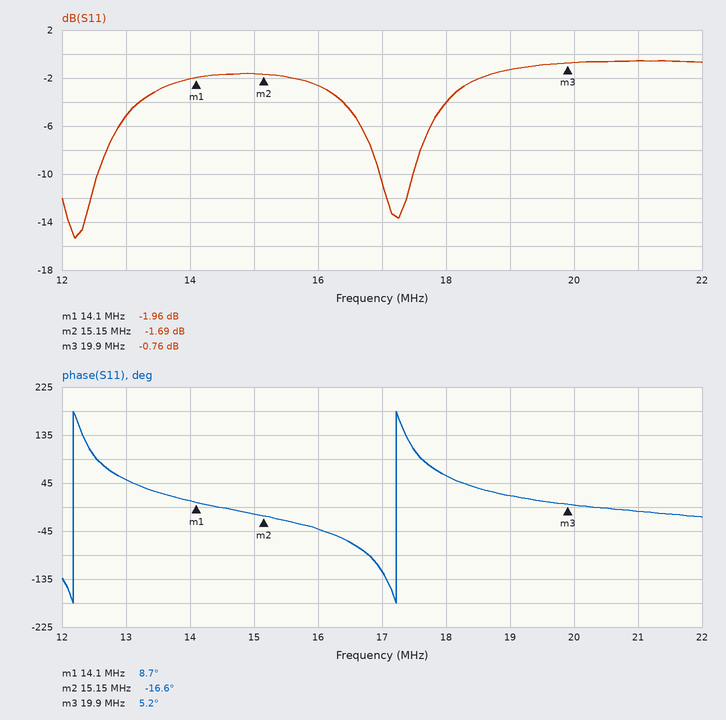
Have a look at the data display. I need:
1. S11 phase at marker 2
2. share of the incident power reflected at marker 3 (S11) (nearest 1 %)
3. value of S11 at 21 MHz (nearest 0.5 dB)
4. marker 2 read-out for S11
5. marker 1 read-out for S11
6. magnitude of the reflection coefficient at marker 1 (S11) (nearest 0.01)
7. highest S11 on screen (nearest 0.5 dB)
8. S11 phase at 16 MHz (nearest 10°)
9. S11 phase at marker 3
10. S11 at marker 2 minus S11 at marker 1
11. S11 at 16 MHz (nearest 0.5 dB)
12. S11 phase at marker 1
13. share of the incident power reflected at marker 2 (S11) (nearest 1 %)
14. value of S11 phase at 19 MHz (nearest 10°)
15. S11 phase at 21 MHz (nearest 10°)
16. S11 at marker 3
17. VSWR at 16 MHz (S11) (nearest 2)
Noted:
-16.6°
84 %
-0.5 dB
-1.69 dB
-1.96 dB
0.80
-0.5 dB
-40°
5.2°
0.27 dB
-2.5 dB
8.7°
68 %
20°
-10°
-0.76 dB
6
